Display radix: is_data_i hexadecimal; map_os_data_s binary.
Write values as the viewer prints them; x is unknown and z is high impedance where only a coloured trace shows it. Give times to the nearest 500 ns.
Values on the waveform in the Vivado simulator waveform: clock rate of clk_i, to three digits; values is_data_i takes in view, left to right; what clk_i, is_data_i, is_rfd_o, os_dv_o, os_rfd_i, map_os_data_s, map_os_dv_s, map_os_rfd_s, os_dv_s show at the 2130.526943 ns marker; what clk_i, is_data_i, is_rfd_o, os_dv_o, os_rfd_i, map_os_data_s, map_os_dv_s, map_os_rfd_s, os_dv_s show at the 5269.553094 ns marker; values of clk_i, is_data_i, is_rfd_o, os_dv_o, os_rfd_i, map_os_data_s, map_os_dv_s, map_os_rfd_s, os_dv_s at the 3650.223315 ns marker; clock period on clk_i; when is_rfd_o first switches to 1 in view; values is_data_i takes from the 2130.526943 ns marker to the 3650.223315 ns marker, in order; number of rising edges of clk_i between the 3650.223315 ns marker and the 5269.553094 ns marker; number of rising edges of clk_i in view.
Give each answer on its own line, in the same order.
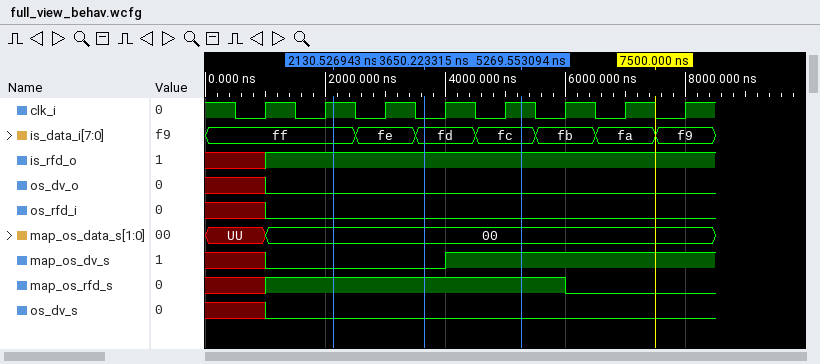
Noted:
1.00 MHz
ff, fe, fd, fc, fb, fa, f9
clk_i=1, is_data_i=ff, is_rfd_o=1, os_dv_o=0, os_rfd_i=0, map_os_data_s=00, map_os_dv_s=0, map_os_rfd_s=1, os_dv_s=0
clk_i=1, is_data_i=fc, is_rfd_o=1, os_dv_o=0, os_rfd_i=0, map_os_data_s=00, map_os_dv_s=1, map_os_rfd_s=1, os_dv_s=0
clk_i=0, is_data_i=fd, is_rfd_o=1, os_dv_o=0, os_rfd_i=0, map_os_data_s=00, map_os_dv_s=0, map_os_rfd_s=1, os_dv_s=0
1000 ns
1000 ns
ff, fe, fd
2
8
